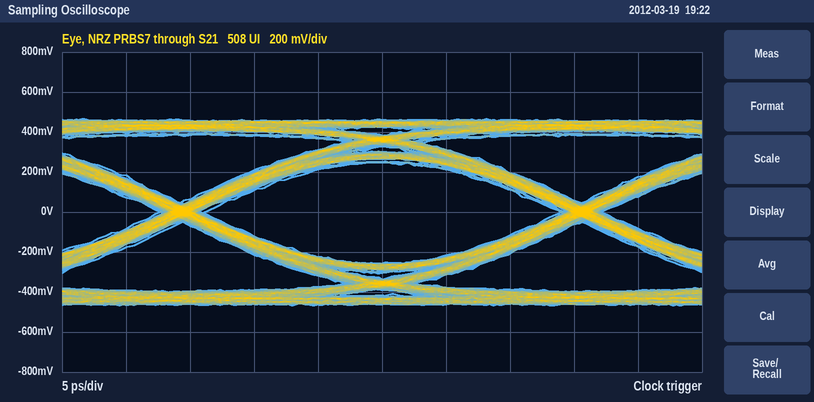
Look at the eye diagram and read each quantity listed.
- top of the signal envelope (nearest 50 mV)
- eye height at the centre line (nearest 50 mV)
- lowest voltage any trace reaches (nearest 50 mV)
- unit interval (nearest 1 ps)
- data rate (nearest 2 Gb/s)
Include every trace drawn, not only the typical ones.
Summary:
450 mV
500 mV
-450 mV
31 ps
32 Gb/s
